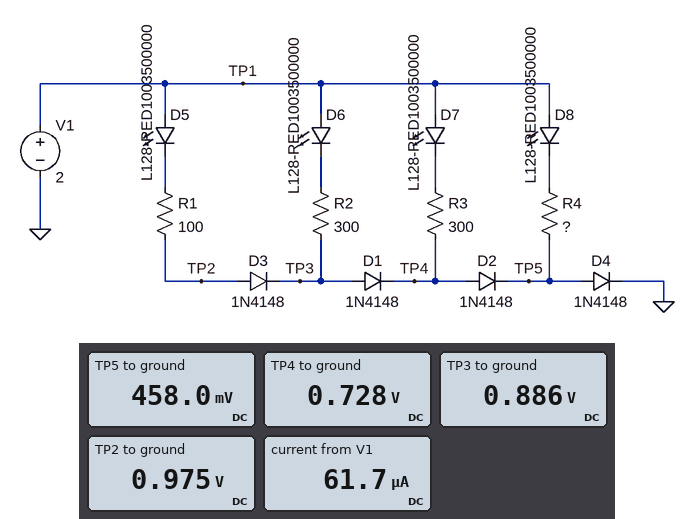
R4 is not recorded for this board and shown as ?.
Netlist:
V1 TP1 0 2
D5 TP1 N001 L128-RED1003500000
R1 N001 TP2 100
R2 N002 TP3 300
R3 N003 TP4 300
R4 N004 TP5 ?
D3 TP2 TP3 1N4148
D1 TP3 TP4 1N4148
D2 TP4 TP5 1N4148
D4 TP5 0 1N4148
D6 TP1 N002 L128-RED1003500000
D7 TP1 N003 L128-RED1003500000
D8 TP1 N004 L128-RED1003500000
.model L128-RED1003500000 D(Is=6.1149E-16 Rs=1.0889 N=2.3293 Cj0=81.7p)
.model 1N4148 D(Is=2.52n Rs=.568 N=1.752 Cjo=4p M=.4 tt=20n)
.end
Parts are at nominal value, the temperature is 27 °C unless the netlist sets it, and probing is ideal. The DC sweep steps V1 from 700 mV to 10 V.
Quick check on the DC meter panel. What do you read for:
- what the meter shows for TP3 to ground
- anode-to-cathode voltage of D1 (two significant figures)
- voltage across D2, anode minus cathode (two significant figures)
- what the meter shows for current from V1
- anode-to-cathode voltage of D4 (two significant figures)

0.886 V
160 mV
270 mV
61.7 µA
460 mV
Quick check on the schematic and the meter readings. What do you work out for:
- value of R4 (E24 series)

270 Ω
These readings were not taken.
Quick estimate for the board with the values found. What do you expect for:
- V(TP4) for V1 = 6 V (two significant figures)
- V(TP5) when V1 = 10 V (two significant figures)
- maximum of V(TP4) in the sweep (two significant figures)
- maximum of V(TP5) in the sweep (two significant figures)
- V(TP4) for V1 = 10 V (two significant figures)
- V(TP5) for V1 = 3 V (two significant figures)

1.5 V
860 mV
1.7 V
860 mV
1.7 V
630 mV
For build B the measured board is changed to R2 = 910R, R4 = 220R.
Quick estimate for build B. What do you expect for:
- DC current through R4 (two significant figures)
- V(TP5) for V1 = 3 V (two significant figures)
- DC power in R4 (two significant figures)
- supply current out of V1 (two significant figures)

62 µA
640 mV
850 nW
63 µA
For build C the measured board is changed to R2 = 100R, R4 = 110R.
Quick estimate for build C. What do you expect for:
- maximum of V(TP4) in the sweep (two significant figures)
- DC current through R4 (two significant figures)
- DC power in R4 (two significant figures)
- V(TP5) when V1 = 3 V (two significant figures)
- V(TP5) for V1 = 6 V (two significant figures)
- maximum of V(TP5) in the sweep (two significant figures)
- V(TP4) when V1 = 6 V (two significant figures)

1.8 V
66 µA
480 nW
660 mV
810 mV
930 mV
1.6 V
